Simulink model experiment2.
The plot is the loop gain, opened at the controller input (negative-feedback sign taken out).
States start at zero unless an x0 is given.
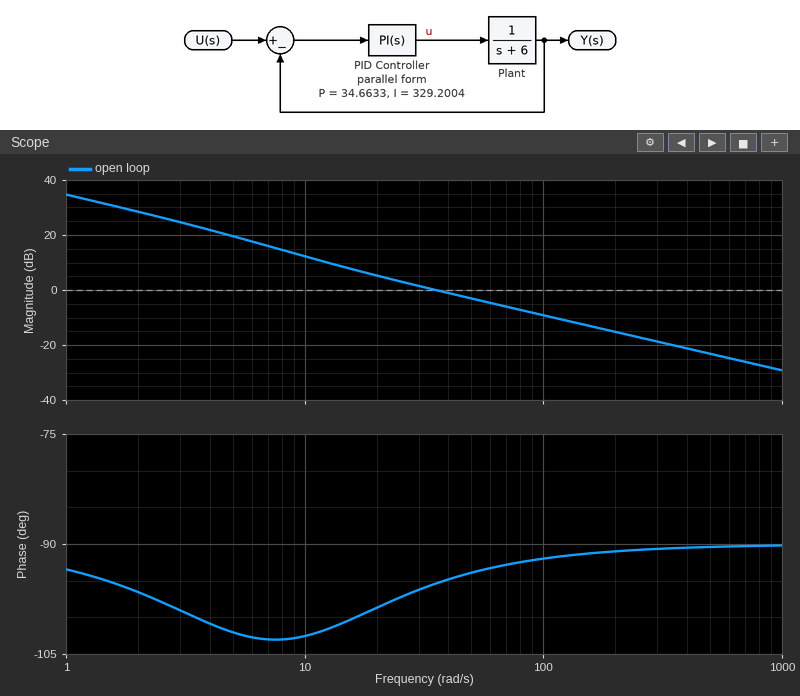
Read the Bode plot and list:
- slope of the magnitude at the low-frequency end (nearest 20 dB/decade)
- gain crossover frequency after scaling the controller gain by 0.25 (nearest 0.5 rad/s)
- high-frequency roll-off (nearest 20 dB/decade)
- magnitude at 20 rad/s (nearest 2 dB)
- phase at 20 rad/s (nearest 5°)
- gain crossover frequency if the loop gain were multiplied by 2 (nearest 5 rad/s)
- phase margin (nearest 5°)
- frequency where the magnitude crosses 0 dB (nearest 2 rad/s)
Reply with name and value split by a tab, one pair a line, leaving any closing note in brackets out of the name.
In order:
slope of the magnitude at the low-frequency end	-20 dB/decade
gain crossover frequency after scaling the controller gain by 0.25	10.0 rad/s
high-frequency roll-off	-20 dB/decade
magnitude at 20 rad/s	6 dB
phase at 20 rad/s	-100°
gain crossover frequency if the loop gain were multiplied by 2	70 rad/s
phase margin	85°
frequency where the magnitude crosses 0 dB	36 rad/s
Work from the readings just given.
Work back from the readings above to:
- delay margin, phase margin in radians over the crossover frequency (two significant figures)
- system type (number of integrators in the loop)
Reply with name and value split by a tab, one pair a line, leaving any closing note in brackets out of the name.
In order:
delay margin, phase margin in radians over the crossover frequency	0.041 s
system type	1
